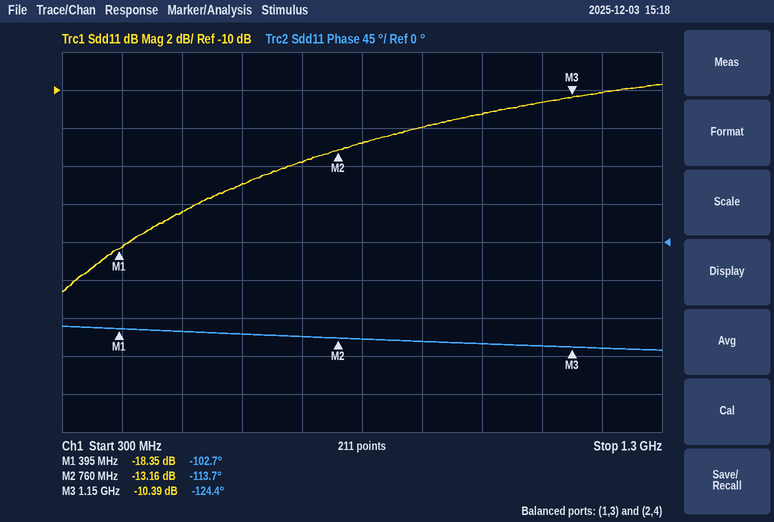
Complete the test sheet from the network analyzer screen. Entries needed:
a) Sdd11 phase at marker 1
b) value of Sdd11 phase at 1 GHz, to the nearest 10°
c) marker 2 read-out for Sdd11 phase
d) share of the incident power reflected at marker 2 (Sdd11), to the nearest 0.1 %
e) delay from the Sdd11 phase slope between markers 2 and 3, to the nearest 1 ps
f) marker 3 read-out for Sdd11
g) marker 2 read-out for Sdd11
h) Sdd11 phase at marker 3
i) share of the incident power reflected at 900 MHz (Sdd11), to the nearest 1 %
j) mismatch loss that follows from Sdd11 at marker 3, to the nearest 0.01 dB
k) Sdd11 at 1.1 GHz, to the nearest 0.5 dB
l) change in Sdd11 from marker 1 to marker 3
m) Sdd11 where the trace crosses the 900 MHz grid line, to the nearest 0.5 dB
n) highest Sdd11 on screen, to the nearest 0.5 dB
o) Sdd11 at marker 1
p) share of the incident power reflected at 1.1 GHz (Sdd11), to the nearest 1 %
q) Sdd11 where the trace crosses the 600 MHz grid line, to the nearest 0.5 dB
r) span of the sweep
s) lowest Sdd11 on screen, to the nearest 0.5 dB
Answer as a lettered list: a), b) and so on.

a) -102.7°
b) -120°
c) -113.7°
d) 4.8 %
e) 76 ps
f) -10.39 dB
g) -13.16 dB
h) -124.4°
i) 6 %
j) 0.42 dB
k) -10.5 dB
l) 7.96 dB
m) -12.0 dB
n) -9.5 dB
o) -18.35 dB
p) 9 %
q) -15.0 dB
r) 1 GHz
s) -20.5 dB
